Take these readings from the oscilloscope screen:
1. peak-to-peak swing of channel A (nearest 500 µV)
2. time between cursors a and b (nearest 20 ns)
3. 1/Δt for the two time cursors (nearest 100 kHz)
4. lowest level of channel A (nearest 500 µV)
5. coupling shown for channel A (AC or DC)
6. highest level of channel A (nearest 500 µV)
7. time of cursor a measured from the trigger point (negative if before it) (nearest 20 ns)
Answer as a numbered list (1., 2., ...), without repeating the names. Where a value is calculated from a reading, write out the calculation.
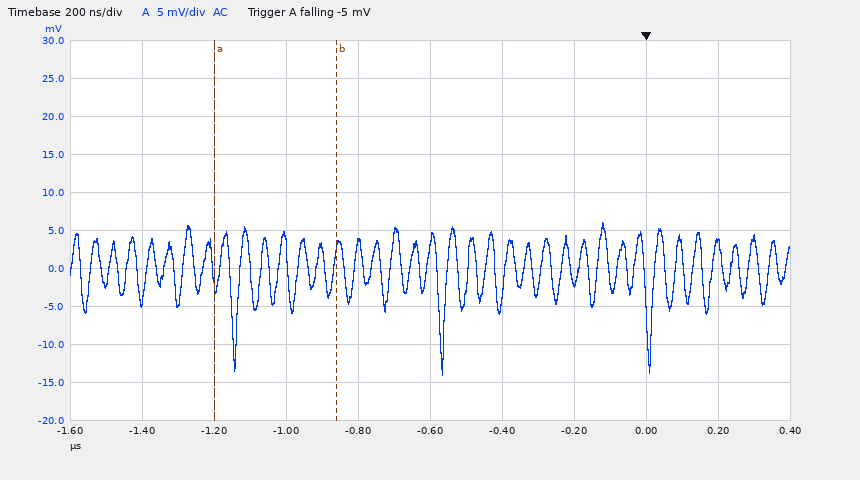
1. 6.0 mV − (-14.0 mV) = 20.0 mV
2. 340 ns
3. 1 / 340 ns ≈ 2.9 MHz
4. -14.0 mV
5. AC
6. 6.0 mV
7. -1.20 µs
